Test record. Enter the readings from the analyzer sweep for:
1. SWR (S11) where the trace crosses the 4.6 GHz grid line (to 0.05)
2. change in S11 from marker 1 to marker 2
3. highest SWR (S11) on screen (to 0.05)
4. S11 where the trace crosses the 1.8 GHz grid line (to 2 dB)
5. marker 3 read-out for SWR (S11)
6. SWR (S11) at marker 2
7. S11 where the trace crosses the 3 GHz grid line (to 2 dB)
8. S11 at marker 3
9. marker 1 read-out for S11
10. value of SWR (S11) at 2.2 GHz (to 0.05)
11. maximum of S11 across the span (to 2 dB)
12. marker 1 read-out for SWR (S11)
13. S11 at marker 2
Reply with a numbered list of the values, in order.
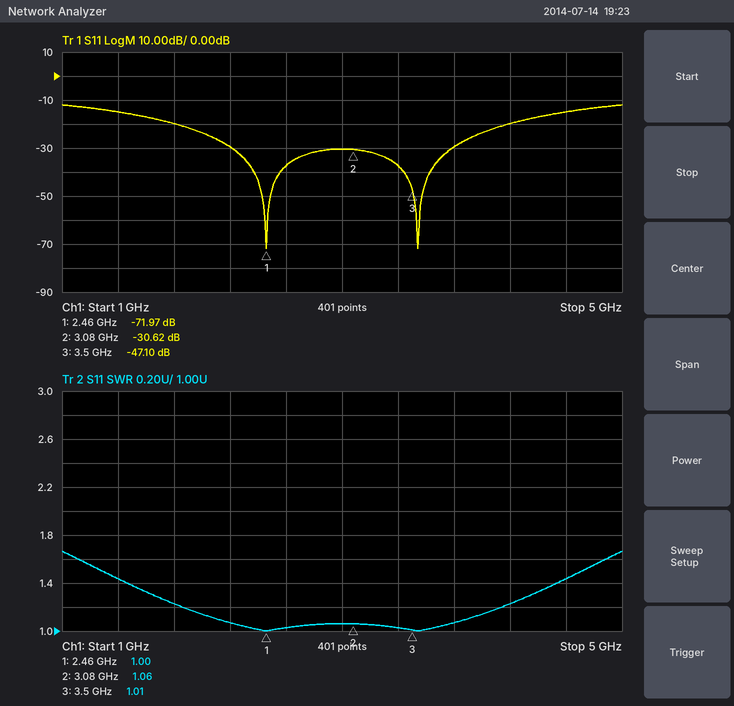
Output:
1. 1.45
2. 41.35 dB
3. 1.65
4. -20 dB
5. 1.01
6. 1.06
7. -30 dB
8. -47.10 dB
9. -71.97 dB
10. 1.05
11. -12 dB
12. 1.00
13. -30.62 dB
